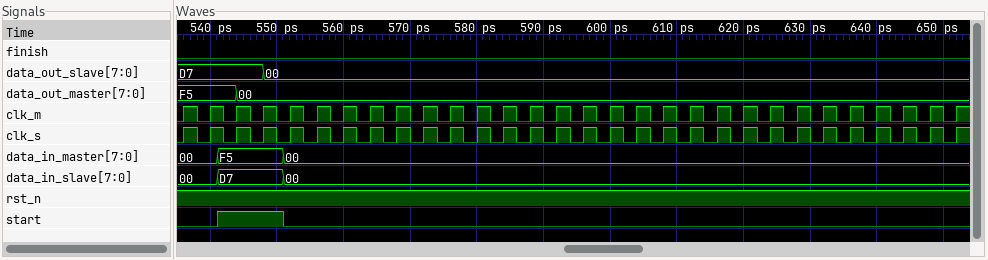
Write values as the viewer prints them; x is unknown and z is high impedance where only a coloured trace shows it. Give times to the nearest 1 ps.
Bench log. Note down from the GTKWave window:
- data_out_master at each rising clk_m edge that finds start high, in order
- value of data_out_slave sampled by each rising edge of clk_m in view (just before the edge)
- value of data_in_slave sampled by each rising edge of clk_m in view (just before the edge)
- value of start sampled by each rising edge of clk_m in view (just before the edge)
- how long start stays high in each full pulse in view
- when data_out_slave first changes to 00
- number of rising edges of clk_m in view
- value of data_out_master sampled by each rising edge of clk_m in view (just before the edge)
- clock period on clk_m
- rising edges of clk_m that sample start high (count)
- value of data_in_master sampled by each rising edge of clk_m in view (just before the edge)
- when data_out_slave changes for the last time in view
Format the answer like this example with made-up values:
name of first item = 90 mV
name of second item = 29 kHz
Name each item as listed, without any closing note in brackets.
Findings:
data_out_master at each rising clk_m edge that finds start high, in order = F5, 00
value of data_out_slave sampled by each rising edge of clk_m in view = D7, D7, D7, D7, 00, 00, 00, 00, 00, 00, 00, 00, 00, 00, 00, 00, 00, 00, 00, 00, 00, 00, 00, 00, 00, 00, 00, 00, 00, 00
value of data_in_slave sampled by each rising edge of clk_m in view = 00, 00, D7, D7, 00, 00, 00, 00, 00, 00, 00, 00, 00, 00, 00, 00, 00, 00, 00, 00, 00, 00, 00, 00, 00, 00, 00, 00, 00, 00
value of start sampled by each rising edge of clk_m in view = 0 0 1 1 0 0 0 0 0 0 0 0 0 0 0 0 0 0 0 0 0 0 0 0 0 0 0 0 0 0
how long start stays high in each full pulse in view = 10 ps
when data_out_slave first changes to 00 = 548 ps
number of rising edges of clk_m in view = 30
value of data_out_master sampled by each rising edge of clk_m in view = F5, F5, F5, 00, 00, 00, 00, 00, 00, 00, 00, 00, 00, 00, 00, 00, 00, 00, 00, 00, 00, 00, 00, 00, 00, 00, 00, 00, 00, 00
clock period on clk_m = 4 ps
rising edges of clk_m that sample start high = 2
value of data_in_master sampled by each rising edge of clk_m in view = 00, 00, F5, F5, 00, 00, 00, 00, 00, 00, 00, 00, 00, 00, 00, 00, 00, 00, 00, 00, 00, 00, 00, 00, 00, 00, 00, 00, 00, 00
when data_out_slave changes for the last time in view = 548 ps
